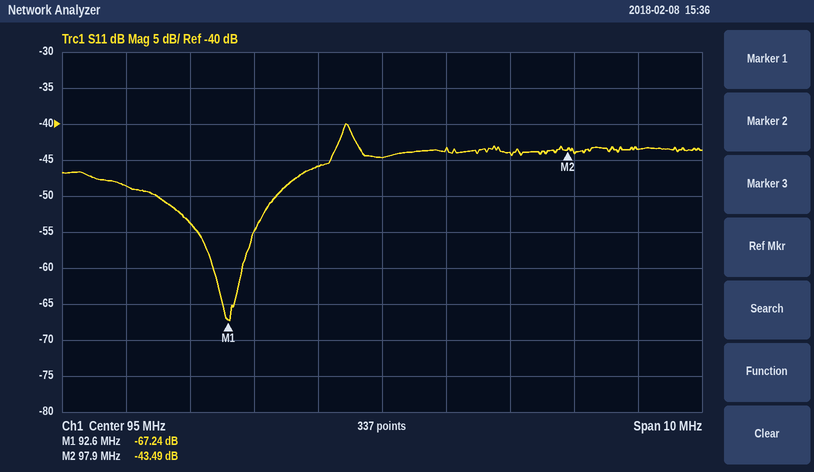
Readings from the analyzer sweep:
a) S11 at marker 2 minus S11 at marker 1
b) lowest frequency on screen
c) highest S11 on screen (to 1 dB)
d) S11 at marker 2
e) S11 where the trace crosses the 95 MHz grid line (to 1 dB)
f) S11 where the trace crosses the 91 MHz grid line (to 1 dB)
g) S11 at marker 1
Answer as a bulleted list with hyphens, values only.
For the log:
- 23.75 dB
- 90 MHz
- -40 dB
- -43.49 dB
- -45 dB
- -49 dB
- -67.24 dB
